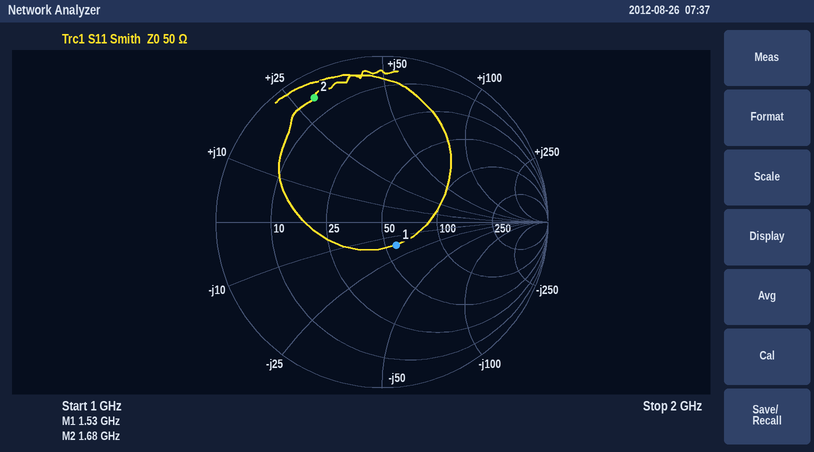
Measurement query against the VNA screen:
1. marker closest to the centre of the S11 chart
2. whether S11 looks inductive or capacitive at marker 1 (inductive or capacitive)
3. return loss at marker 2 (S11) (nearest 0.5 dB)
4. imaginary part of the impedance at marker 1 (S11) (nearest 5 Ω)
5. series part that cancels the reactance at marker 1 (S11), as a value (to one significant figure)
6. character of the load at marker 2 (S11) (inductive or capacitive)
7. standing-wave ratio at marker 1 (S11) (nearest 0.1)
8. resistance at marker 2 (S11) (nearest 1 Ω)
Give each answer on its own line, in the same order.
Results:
marker 1
capacitive
1.5 dB
-15 Ω
2 nH
inductive
1.4
5 Ω
